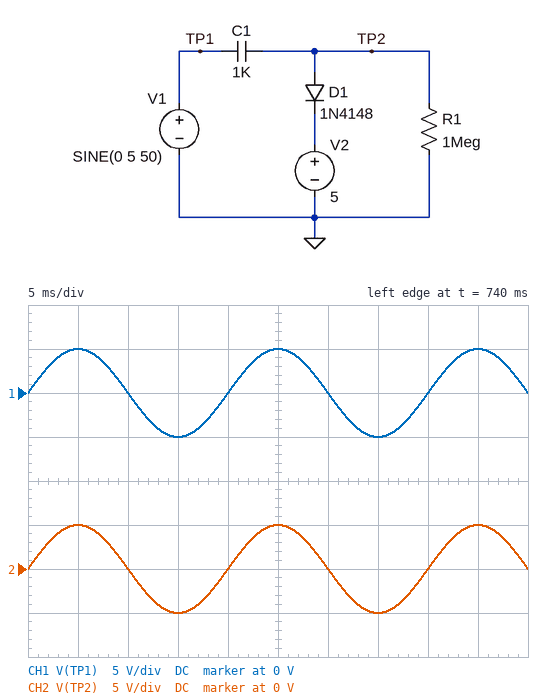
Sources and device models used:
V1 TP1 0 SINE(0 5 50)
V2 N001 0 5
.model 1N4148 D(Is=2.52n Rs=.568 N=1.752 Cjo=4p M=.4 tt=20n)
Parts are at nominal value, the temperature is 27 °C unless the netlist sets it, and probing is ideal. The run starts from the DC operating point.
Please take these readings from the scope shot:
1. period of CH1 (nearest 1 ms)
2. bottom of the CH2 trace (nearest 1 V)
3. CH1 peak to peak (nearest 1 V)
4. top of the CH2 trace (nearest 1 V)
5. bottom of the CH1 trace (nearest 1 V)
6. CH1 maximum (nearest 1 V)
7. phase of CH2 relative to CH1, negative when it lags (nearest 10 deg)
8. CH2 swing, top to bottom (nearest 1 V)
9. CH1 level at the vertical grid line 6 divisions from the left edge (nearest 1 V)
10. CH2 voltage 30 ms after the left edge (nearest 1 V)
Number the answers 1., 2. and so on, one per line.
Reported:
1. 20 ms
2. -5 V
3. 10 V
4. 5 V
5. -5 V
6. 5 V
7. 0 deg
8. 10 V
9. 0 V
10. 0 V
